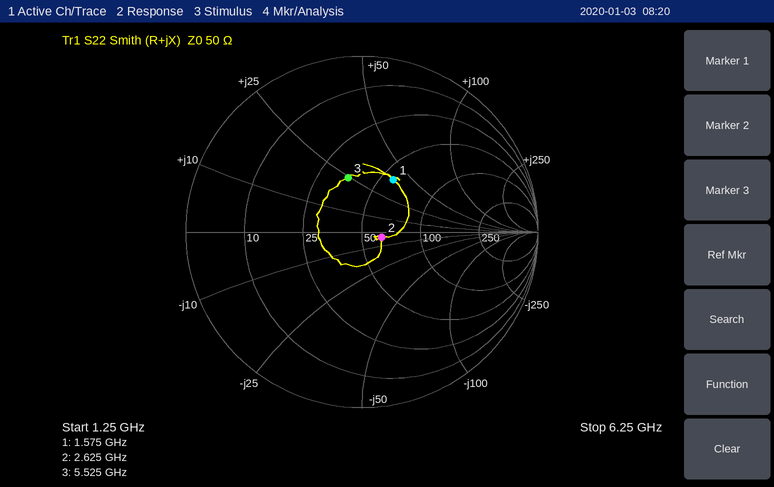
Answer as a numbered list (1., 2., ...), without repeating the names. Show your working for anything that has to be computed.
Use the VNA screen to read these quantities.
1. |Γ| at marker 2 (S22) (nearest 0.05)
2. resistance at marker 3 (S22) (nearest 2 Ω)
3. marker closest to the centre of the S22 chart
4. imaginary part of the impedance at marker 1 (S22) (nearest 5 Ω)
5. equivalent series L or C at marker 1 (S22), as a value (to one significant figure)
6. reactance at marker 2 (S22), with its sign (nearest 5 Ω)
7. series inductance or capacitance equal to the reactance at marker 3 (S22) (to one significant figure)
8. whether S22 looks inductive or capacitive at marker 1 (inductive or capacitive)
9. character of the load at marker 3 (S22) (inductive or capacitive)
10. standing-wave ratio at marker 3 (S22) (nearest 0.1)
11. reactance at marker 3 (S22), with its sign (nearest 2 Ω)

1. 0.10
2. 36 Ω
3. marker 2
4. +40 Ω
5. L = 40 Ω/(2π × 1.575 GHz) ≈ 4 nH
6. -5 Ω
7. L = 24 Ω/(2π × 5.525 GHz) ≈ 691 pH, so 700 pH to one significant figure
8. inductive
9. inductive
10. 1.9
11. +24 Ω
